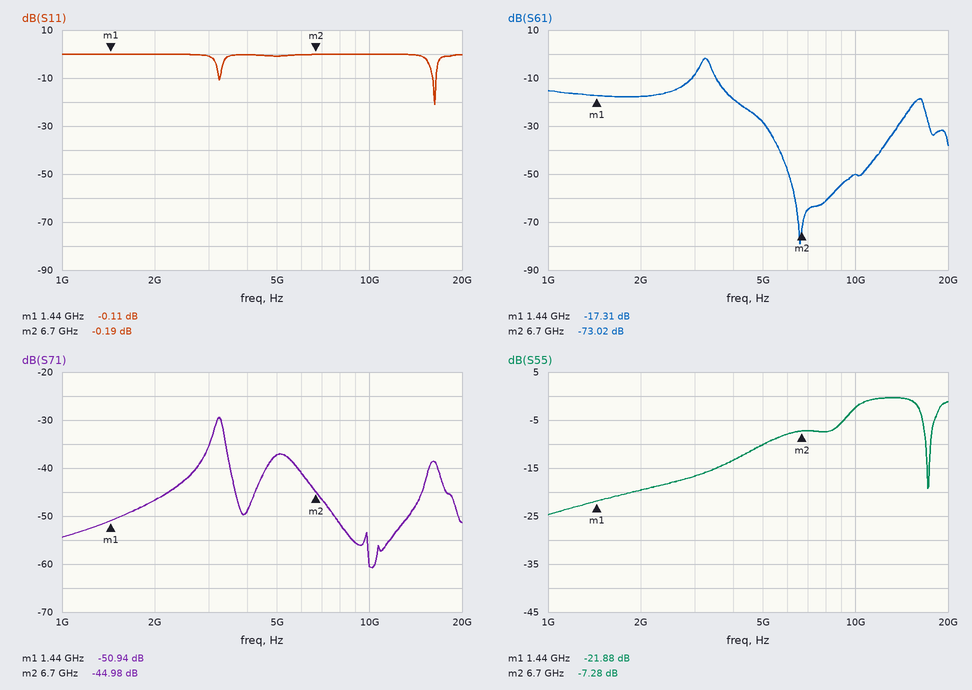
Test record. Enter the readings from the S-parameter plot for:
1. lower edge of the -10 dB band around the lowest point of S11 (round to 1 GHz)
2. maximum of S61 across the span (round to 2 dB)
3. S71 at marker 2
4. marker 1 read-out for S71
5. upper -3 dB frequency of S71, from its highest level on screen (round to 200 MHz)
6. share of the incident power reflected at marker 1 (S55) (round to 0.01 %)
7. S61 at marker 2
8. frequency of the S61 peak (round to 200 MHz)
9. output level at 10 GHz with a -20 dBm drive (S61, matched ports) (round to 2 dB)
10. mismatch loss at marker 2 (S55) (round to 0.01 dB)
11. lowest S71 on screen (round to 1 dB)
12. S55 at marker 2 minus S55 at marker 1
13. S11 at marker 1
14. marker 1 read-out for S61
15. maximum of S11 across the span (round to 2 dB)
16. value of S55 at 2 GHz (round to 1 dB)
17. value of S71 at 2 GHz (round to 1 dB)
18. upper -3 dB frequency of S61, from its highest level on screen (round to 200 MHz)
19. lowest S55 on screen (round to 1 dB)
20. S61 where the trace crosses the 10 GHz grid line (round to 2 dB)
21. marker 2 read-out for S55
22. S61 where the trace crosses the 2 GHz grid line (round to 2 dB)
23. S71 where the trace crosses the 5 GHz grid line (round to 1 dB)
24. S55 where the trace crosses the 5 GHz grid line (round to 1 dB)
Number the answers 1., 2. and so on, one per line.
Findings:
1. 16 GHz
2. -2 dB
3. -44.98 dB
4. -50.94 dB
5. 3.4 GHz
6. 0.65 %
7. -73.02 dB
8. 3.2 GHz
9. -70 dBm
10. 0.90 dB
11. -61 dB
12. 14.60 dB
13. -0.11 dB
14. -17.31 dB
15. 0 dB
16. -20 dB
17. -47 dB
18. 3.4 GHz
19. -25 dB
20. -50 dB
21. -7.28 dB
22. -18 dB
23. -37 dB
24. -10 dB
